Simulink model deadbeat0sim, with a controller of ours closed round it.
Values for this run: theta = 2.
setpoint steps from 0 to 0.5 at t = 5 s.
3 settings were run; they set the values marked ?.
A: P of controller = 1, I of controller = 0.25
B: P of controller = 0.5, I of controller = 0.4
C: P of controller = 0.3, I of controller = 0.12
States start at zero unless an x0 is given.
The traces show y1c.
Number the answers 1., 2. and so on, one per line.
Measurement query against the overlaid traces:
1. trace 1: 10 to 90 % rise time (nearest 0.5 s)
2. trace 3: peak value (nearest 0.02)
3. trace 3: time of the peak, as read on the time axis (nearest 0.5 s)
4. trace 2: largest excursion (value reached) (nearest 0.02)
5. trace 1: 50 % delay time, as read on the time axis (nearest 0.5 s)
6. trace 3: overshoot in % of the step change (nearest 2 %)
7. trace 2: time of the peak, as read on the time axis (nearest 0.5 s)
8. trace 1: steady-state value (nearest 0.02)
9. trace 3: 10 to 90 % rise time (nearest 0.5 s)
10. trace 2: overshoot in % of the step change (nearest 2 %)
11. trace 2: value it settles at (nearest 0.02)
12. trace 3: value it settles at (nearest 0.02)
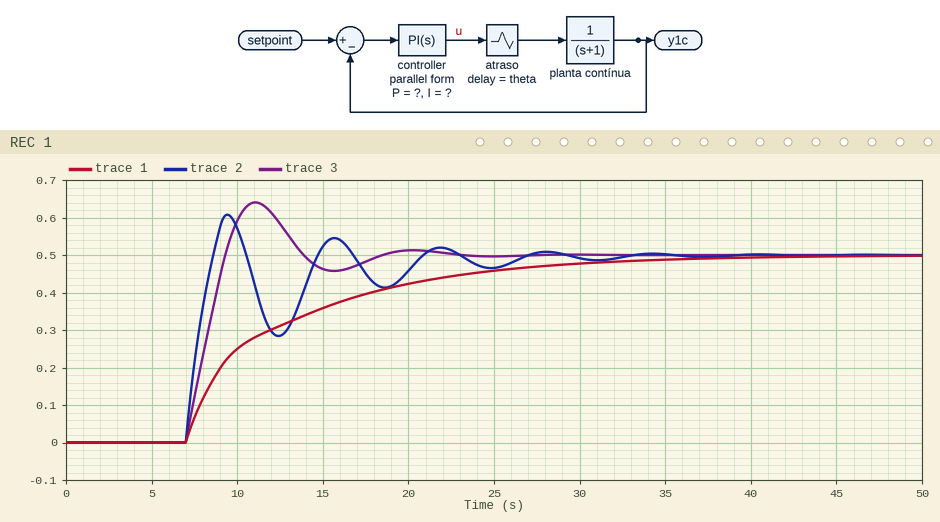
1. 16.0 s
2. 0.64
3. 11.0 s
4. 0.60
5. 10.0 s
6. 28 %
7. 9.5 s
8. 0.50
9. 2.0 s
10. 22 %
11. 0.50
12. 0.50
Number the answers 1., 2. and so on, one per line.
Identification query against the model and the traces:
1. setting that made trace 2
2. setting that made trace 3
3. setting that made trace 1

1. A
2. B
3. C
